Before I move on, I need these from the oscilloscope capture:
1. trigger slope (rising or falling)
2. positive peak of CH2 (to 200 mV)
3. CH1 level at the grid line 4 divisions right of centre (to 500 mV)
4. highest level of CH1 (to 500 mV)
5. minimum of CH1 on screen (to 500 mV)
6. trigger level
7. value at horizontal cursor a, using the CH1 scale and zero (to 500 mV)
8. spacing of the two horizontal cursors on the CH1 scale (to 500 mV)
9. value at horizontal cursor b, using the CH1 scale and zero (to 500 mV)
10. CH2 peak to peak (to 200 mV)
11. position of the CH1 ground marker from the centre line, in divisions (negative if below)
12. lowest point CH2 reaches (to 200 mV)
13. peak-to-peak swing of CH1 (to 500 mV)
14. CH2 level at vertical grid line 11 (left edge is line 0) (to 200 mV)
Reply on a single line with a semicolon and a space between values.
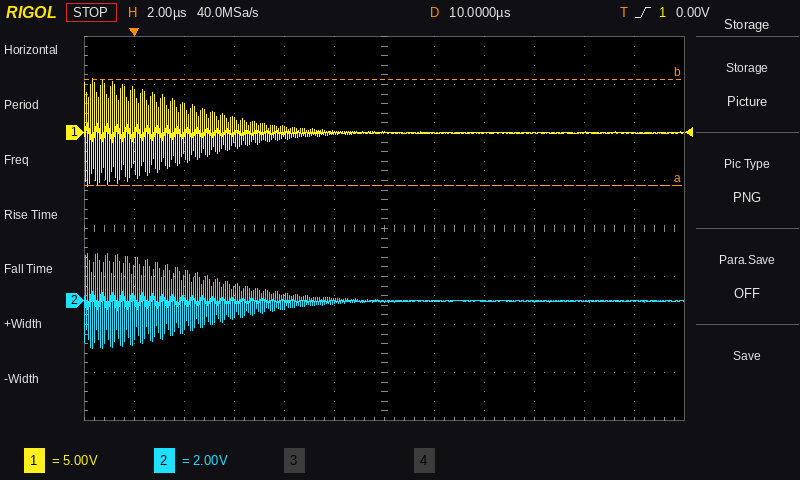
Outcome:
rising; 2.0 V; 0.0 V; 5.5 V; -5.5 V; 0.00 V; -5.5 V; 11.0 V; 5.5 V; 4.0 V; +2.0 div; -2.0 V; 11.0 V; 0.0 V
